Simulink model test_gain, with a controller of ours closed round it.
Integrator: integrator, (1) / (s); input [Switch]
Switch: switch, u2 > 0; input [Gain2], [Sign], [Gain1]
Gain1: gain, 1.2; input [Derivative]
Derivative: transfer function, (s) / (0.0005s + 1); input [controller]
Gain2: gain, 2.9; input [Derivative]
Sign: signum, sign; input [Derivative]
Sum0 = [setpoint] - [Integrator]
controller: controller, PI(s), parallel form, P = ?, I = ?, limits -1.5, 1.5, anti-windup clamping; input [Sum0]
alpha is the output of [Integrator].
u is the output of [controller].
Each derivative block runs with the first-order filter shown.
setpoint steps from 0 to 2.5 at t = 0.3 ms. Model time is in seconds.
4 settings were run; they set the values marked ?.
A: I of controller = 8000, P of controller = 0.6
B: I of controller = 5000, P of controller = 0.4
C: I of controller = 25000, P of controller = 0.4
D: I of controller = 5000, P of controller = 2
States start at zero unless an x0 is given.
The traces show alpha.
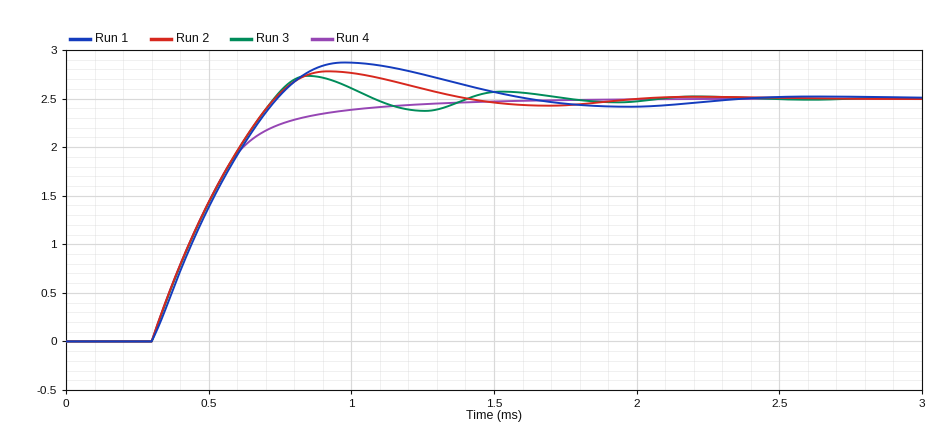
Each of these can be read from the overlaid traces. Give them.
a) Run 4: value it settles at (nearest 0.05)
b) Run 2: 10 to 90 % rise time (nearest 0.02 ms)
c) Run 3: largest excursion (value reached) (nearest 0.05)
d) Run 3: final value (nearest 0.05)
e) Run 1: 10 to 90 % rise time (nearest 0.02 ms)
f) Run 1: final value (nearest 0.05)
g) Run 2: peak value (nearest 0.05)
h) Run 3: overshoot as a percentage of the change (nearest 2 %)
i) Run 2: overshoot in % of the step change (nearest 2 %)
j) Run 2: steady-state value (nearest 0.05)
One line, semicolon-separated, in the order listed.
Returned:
2.50; 0.34 ms; 2.75; 2.50; 0.34 ms; 2.50; 2.80; 10 %; 12 %; 2.50
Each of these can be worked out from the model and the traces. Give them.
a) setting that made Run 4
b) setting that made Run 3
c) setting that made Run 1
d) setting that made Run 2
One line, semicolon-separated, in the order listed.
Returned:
D; C; B; A
